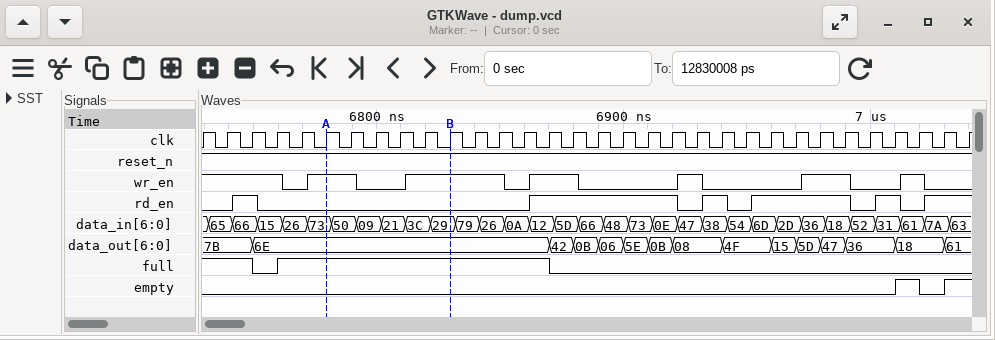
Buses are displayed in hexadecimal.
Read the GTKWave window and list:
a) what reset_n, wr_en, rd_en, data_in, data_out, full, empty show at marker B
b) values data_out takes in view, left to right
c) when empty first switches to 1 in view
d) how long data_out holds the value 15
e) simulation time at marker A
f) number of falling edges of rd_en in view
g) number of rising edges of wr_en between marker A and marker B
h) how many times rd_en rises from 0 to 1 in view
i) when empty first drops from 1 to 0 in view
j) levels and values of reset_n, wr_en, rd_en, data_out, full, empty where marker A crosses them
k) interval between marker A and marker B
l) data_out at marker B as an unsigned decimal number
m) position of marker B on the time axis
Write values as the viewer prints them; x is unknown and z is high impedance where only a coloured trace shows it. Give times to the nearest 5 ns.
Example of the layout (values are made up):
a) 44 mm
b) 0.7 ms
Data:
a) reset_n=1, wr_en=1, rd_en=0, data_in=29, data_out=6E, full=1, empty=0
b) 7B, 6E, 42, 0B, 06, 5E, 0B, 08, 4F, 15, 5D, 47, 36, 18, 61
c) 7010 ns
d) 10 ns
e) 6780 ns
f) 5
g) 1
h) 6
i) 7020 ns
j) reset_n=1, wr_en=1, rd_en=0, data_out=6E, full=1, empty=0
k) 50 ns
l) 110
m) 6830 ns
